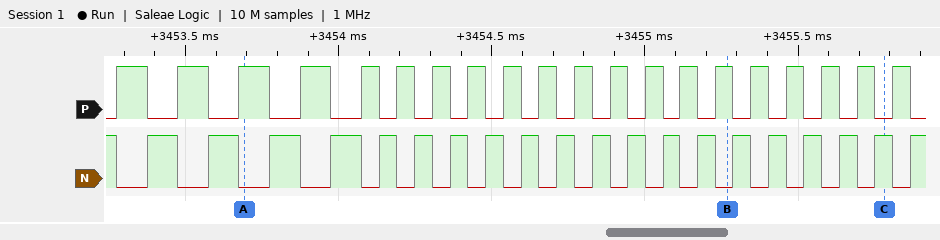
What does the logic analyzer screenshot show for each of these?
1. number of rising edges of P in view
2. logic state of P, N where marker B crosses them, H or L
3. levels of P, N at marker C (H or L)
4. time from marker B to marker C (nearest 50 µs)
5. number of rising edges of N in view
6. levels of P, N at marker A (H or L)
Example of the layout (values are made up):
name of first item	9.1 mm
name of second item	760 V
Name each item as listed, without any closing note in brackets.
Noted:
number of rising edges of P in view	20
logic state of P, N where marker B crosses them, H or L	P=H, N=L
levels of P, N at marker C	P=L, N=H
time from marker B to marker C	500 µs
number of rising edges of N in view	20
levels of P, N at marker A	P=H, N=L
